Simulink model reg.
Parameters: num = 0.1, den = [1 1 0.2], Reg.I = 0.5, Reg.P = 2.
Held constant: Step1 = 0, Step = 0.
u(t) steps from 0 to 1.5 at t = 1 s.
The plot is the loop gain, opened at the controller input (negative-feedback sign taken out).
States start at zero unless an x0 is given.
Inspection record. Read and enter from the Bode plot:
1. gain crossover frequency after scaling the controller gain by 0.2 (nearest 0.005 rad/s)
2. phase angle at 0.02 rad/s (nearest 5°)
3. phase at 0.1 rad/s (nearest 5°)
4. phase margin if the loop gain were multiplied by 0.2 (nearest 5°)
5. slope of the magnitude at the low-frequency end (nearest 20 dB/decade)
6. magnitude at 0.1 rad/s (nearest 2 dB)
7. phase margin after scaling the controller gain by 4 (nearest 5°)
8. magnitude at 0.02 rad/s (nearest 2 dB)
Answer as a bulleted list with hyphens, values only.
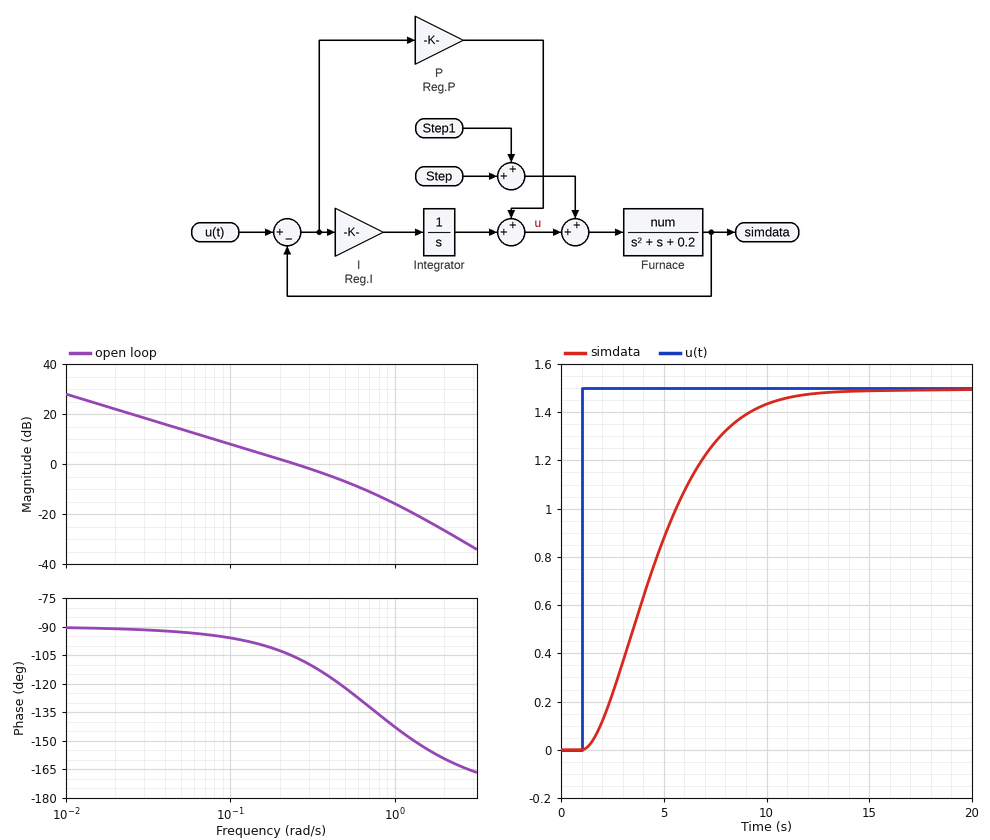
- 0.050 rad/s
- -90°
- -95°
- 85°
- -20 dB/decade
- 8 dB
- 45°
- 22 dB
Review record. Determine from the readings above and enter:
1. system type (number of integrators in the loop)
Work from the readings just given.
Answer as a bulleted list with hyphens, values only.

- 1
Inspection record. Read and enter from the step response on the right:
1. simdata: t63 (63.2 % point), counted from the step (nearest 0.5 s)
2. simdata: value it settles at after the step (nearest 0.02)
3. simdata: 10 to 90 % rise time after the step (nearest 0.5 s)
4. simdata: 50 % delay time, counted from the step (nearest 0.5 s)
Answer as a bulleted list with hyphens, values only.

- 4.5 s
- 1.50
- 6.0 s
- 3.5 s
